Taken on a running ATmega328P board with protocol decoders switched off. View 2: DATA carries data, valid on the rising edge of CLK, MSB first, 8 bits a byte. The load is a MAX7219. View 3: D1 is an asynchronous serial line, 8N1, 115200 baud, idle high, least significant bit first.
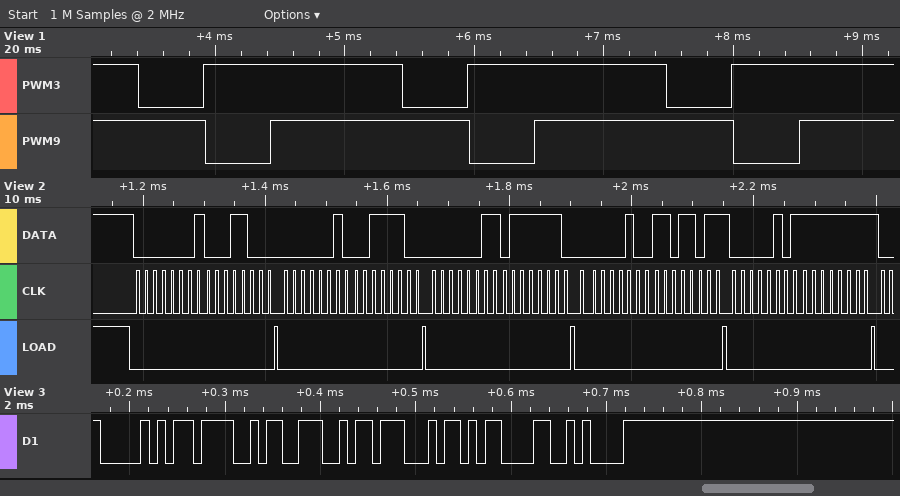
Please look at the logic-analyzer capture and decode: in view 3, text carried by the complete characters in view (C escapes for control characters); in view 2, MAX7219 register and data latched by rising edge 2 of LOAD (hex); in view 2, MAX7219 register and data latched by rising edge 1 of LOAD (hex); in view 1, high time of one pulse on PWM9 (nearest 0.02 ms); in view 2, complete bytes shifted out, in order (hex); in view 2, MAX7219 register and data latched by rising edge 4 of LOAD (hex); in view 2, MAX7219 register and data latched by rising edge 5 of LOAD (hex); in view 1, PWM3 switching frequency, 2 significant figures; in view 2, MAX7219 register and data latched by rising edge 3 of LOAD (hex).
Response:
"PONG\r\n"
register 0x2, data 0x3C
register 0x1, data 0x18
1.54 ms
01 18 02 3C 03 7E 04 DB 05 FF
register 0x4, data 0xDB
register 0x5, data 0xFF
490 Hz
register 0x3, data 0x7E
